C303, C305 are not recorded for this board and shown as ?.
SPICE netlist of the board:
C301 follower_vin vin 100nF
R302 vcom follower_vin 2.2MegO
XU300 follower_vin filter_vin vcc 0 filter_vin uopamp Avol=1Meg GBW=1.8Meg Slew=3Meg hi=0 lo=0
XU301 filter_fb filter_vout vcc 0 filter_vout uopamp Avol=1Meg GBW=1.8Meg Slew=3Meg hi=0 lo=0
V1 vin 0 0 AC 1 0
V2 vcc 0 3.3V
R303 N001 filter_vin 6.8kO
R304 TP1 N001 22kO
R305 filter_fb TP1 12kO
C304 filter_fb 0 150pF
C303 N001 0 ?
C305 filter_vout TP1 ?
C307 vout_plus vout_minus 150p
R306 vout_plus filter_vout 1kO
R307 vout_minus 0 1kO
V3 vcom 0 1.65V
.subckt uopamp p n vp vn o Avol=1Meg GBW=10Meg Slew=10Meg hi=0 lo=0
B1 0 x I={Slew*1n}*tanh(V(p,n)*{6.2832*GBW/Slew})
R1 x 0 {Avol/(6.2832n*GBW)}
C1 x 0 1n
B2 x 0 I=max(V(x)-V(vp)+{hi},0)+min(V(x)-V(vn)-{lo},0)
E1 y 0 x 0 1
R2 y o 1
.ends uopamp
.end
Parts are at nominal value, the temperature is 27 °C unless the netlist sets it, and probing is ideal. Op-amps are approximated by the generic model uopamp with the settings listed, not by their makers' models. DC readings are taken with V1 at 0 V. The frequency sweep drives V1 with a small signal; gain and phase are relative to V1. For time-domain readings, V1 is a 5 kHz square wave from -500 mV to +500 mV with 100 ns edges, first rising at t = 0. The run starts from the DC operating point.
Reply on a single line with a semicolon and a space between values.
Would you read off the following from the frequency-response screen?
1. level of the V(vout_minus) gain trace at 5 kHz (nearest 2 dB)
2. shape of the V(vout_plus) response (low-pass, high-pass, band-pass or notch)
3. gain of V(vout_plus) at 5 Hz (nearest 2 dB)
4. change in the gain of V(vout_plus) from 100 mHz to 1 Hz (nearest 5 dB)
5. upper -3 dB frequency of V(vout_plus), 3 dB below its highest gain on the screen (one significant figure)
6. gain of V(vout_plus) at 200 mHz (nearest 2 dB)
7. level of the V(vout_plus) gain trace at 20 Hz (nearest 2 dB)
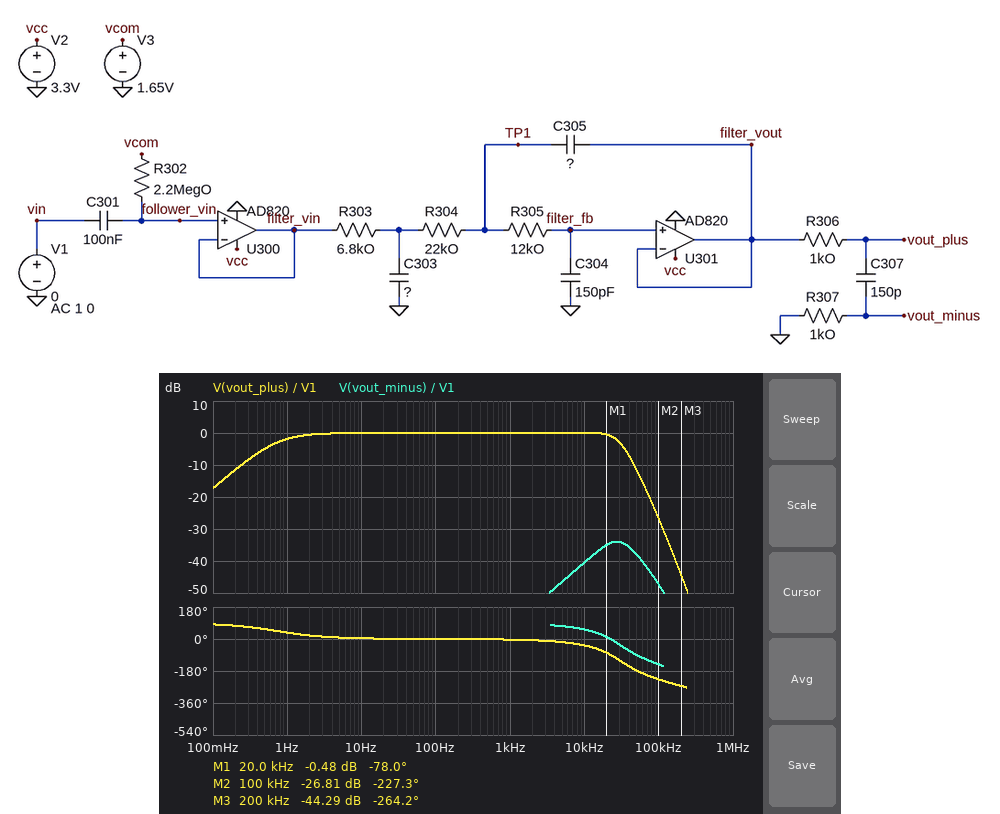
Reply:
-46 dB; band-pass; 0 dB; 15 dB; 30 kHz; -12 dB; 0 dB
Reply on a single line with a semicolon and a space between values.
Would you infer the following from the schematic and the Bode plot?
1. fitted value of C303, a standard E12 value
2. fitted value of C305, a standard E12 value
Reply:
470 pF; 560 pF
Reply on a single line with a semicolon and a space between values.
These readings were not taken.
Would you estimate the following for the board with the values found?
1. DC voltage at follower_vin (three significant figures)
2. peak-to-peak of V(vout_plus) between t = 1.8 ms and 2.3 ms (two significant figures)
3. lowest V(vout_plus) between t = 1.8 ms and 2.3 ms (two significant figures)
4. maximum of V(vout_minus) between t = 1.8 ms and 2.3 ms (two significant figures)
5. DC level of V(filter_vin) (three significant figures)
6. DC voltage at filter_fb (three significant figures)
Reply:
1.65 V; 1.1 V; 1.6 V; 12 mV; 1.65 V; 1.65 V
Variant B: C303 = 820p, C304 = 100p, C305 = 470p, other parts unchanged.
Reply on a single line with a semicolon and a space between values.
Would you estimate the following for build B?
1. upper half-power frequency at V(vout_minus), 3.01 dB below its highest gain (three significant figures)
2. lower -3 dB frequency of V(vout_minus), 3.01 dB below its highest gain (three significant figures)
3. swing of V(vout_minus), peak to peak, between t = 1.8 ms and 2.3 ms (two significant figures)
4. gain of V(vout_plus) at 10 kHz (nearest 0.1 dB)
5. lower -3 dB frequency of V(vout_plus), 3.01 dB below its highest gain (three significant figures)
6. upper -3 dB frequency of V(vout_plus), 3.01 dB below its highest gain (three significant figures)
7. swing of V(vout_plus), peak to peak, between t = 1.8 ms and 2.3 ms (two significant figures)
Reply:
55.4 kHz; 18.0 kHz; 26 mV; -0.3 dB; 723 mHz; 31.8 kHz; 1.0 V
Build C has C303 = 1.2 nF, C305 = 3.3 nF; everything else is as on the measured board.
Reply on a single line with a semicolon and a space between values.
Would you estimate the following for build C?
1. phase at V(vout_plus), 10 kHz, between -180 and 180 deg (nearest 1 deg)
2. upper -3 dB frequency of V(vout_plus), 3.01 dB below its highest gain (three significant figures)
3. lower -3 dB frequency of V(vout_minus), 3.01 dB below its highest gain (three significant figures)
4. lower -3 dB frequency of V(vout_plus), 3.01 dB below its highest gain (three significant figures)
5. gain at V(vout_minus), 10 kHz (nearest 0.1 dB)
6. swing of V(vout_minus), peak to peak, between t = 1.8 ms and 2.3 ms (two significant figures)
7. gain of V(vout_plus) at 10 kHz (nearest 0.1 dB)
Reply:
-80 deg; 14.1 kHz; 8.86 kHz; 5.17 kHz; -36.5 dB; 13 mV; 4.0 dB
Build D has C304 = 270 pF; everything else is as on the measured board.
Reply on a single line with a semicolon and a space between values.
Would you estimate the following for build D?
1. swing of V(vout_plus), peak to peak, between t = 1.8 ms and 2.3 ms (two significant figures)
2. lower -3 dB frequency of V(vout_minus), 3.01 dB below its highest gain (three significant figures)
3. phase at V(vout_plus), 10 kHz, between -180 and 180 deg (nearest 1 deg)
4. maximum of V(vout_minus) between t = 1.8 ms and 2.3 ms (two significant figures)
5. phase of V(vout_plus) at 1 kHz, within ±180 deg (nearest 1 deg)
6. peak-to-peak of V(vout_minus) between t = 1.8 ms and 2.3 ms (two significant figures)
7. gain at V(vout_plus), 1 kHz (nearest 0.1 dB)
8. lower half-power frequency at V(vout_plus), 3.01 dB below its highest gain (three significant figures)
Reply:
1.0 V; 9.89 kHz; -53 deg; 8.1 mV; -5 deg; 16 mV; 0 dB; 723 mHz
